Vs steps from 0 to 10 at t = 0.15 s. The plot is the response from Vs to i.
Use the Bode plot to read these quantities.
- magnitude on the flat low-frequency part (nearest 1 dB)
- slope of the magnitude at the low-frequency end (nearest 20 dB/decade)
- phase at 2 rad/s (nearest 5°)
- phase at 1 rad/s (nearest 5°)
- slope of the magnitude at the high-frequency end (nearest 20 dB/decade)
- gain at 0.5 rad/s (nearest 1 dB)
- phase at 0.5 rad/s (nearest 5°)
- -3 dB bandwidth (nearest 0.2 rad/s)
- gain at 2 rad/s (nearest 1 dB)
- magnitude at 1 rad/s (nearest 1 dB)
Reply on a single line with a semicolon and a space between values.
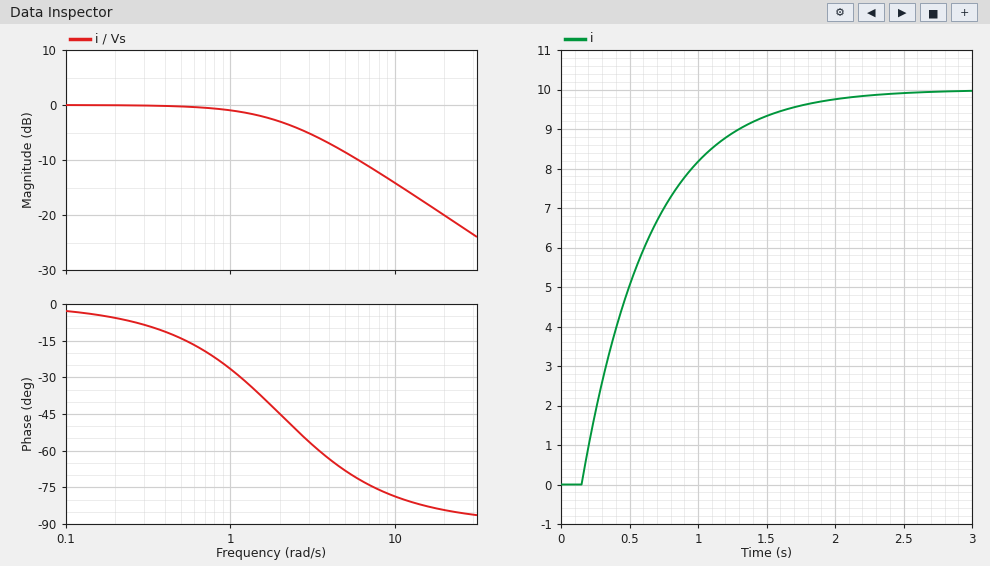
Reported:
0 dB; 0 dB/decade; -45°; -25°; -20 dB/decade; 0 dB; -15°; 2.0 rad/s; -3 dB; -1 dB
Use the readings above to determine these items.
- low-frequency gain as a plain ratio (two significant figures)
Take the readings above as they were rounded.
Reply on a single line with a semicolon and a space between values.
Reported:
1.0
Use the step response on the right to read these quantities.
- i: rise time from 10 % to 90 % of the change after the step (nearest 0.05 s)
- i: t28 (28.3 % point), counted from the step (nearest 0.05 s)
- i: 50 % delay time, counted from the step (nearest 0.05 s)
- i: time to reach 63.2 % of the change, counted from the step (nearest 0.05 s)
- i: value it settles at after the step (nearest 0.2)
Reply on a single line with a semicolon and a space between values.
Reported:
1.10 s; 0.15 s; 0.35 s; 0.50 s; 10.0
